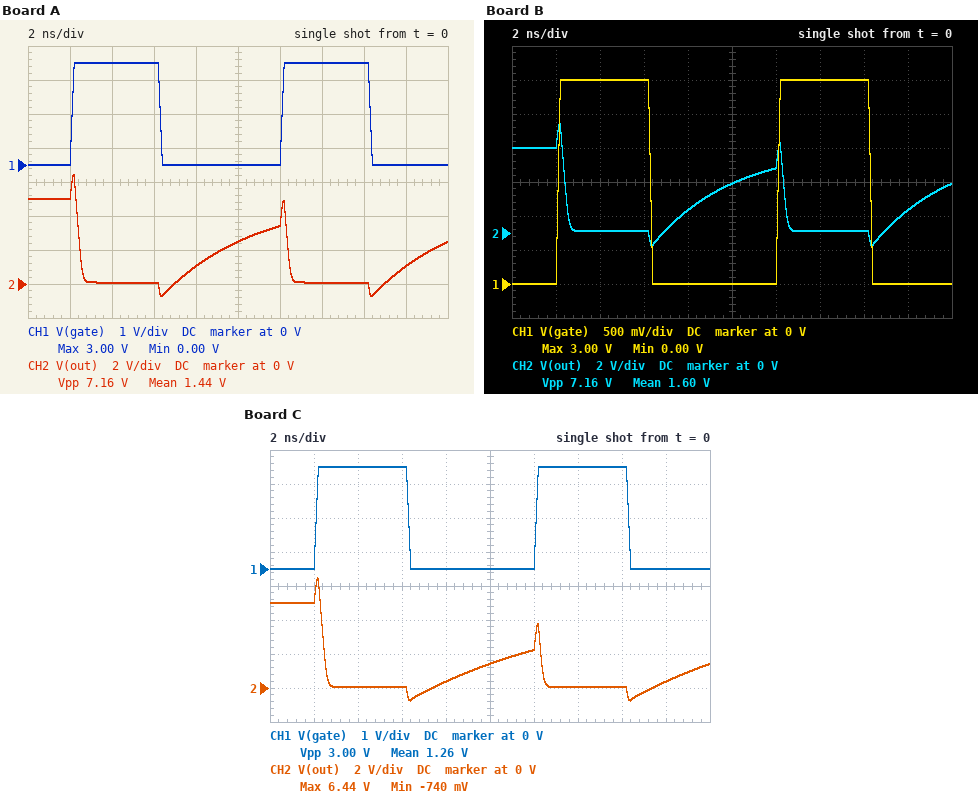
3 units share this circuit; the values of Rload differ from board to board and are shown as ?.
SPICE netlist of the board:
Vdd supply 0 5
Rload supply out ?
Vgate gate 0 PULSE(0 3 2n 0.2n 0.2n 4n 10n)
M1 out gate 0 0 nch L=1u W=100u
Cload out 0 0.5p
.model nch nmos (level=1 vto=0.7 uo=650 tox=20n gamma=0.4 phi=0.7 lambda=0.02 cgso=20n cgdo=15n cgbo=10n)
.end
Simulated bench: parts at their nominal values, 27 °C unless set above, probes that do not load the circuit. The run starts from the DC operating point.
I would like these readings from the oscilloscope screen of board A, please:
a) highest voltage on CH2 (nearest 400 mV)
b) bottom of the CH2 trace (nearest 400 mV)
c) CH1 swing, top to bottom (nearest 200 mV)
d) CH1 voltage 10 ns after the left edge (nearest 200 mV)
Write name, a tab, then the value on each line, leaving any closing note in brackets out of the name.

highest voltage on CH2	6.4 V
bottom of the CH2 trace	-800 mV
CH1 swing, top to bottom	3.0 V
CH1 voltage 10 ns after the left edge	0 V
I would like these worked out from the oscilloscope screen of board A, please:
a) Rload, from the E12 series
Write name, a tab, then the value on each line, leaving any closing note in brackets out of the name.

Rload, from the E12 series	2.2 kΩ
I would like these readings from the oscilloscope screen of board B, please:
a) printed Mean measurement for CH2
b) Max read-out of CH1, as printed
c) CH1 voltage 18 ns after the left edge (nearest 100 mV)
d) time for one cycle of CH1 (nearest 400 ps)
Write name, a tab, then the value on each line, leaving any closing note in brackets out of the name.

printed Mean measurement for CH2	1.60 V
Max read-out of CH1, as printed	3.00 V
CH1 voltage 18 ns after the left edge	0 V
time for one cycle of CH1	10.0 ns
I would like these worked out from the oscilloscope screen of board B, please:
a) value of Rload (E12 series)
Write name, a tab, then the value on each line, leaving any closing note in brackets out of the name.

value of Rload	1.8 kΩ
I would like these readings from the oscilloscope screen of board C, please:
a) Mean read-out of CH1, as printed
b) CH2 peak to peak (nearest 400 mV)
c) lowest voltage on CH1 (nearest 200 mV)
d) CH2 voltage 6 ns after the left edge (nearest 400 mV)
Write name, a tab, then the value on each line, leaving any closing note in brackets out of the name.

Mean read-out of CH1, as printed	1.26 V
CH2 peak to peak	7.2 V
lowest voltage on CH1	0 V
CH2 voltage 6 ns after the left edge	0 V
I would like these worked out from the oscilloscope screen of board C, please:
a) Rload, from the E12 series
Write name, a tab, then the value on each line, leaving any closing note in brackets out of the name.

Rload, from the E12 series	3.9 kΩ
